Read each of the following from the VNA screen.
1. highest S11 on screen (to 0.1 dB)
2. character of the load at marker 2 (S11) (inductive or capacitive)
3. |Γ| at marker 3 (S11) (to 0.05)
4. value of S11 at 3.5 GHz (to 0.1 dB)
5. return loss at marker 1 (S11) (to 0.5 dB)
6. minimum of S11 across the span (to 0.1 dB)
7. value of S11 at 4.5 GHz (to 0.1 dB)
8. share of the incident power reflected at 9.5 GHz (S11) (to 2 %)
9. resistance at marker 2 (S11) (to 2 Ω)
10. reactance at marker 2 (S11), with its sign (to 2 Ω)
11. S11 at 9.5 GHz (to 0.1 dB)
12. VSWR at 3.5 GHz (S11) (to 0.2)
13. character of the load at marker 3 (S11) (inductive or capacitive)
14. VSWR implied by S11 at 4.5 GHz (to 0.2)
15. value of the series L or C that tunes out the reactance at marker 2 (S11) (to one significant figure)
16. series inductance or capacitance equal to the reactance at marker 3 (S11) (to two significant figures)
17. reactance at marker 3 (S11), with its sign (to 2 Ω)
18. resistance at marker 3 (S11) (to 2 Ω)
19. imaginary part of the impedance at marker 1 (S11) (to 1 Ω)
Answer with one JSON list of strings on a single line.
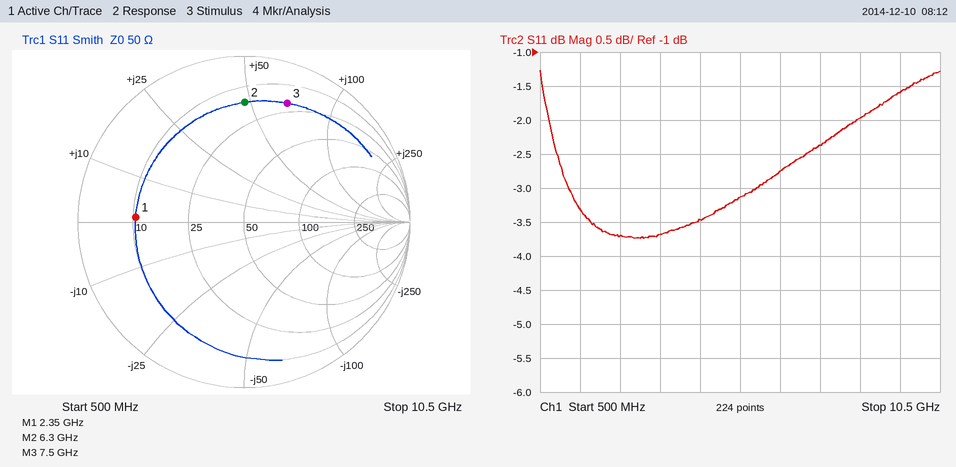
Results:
["-1.3 dB", "inductive", "0.75", "-3.7 dB", "3.5 dB", "-3.7 dB", "-3.5 dB", "70 %", "16 Ω", "+48 Ω", "-1.6 dB", "4.8", "inductive", "5.0", "500 fF", "1.4 nH", "+68 Ω", "20 Ω", "+1 Ω"]
